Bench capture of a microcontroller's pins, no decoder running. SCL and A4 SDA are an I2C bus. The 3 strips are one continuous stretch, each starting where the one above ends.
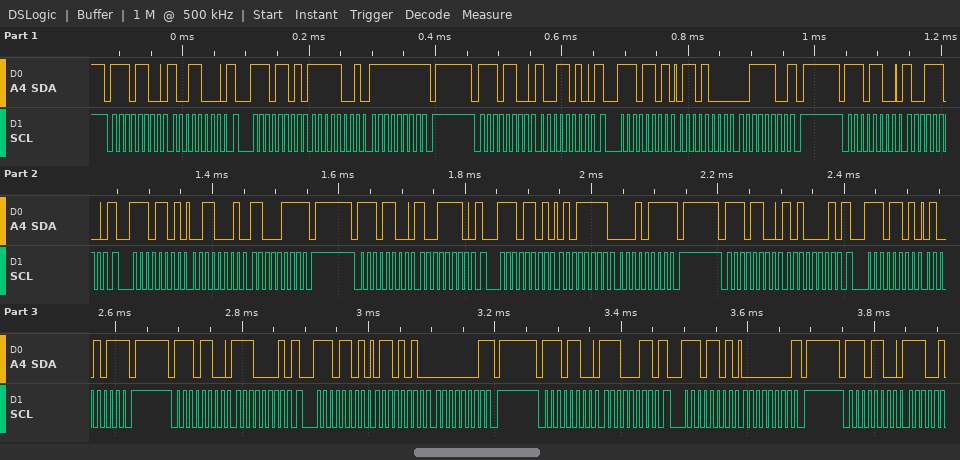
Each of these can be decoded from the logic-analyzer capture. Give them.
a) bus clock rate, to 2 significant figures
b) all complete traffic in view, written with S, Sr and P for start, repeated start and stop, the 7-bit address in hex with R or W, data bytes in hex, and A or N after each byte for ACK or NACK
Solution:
100 kHz
S 76W A 98 A Sr 76R A F9 A FF N P S 76W A 9A A Sr 76R A 68 A 3C N P S 76W A 9C A Sr 76R A 31 A C7 N P S 76W A 9E A Sr 76R A 5F A 17 N P S 76W A A1 A Sr 76R A 4B N P S 76W A E1 A Sr 76R A 6A A 01 N P S 76W A E3 A Sr 76R A 00 N P S 76W A
